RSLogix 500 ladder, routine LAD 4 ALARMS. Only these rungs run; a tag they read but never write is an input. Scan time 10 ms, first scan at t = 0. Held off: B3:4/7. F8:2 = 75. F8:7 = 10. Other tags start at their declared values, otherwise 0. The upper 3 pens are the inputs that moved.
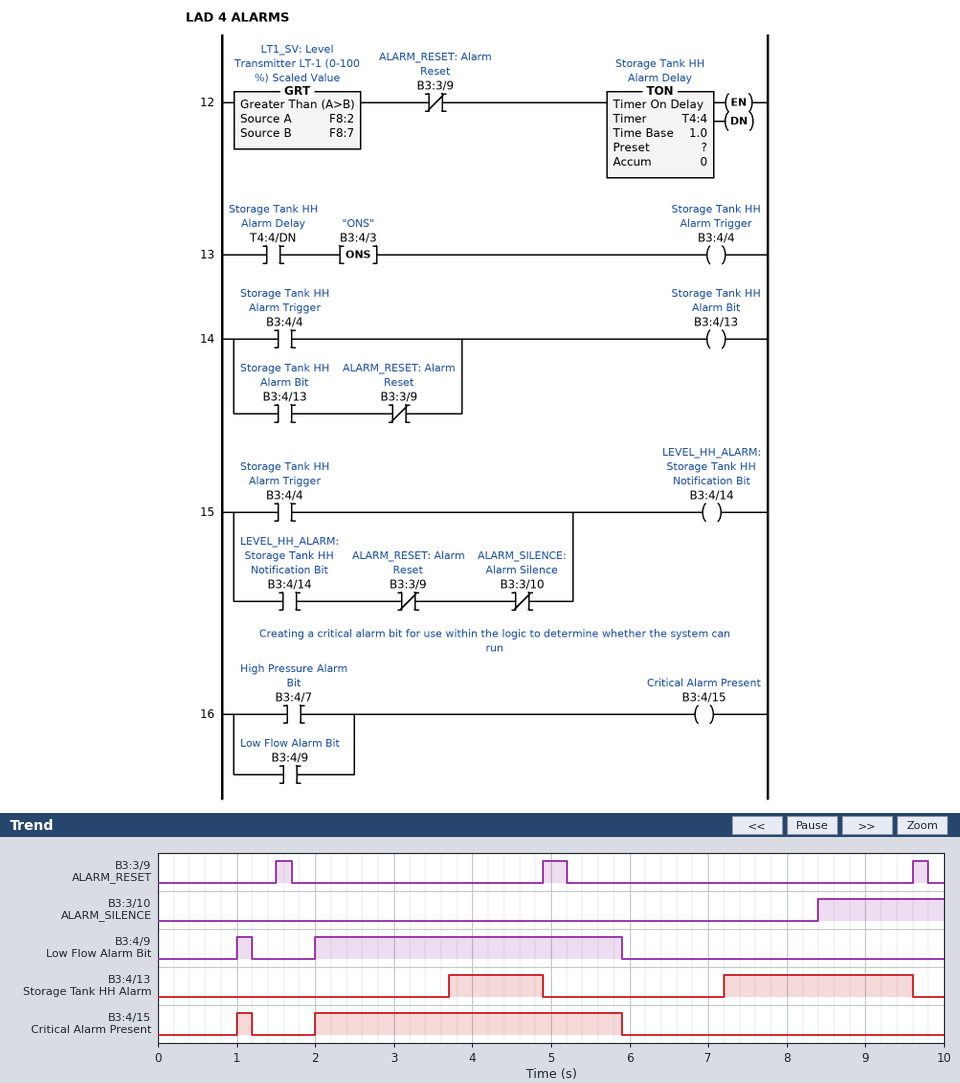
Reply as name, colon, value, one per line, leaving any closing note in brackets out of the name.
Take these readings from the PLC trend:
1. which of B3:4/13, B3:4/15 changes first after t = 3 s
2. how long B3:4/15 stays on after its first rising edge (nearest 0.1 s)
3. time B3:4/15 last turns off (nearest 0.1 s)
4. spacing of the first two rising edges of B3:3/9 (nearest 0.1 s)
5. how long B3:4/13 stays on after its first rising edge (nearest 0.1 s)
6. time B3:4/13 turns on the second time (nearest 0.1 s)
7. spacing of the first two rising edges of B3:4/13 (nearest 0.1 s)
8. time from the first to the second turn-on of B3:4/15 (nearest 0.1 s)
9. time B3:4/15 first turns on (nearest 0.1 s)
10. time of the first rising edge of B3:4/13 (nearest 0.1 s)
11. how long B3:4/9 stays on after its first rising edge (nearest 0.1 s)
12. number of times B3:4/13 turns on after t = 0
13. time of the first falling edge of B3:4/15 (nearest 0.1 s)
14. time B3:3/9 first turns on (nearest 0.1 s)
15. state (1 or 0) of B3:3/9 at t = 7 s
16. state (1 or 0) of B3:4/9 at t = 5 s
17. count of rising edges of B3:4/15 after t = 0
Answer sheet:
which of B3:4/13, B3:4/15 changes first after t = 3 s: B3:4/13
how long B3:4/15 stays on after its first rising edge: 0.2 s
time B3:4/15 last turns off: 5.9 s
spacing of the first two rising edges of B3:3/9: 3.4 s
how long B3:4/13 stays on after its first rising edge: 1.2 s
time B3:4/13 turns on the second time: 7.2 s
spacing of the first two rising edges of B3:4/13: 3.5 s
time from the first to the second turn-on of B3:4/15: 1.0 s
time B3:4/15 first turns on: 1.0 s
time of the first rising edge of B3:4/13: 3.7 s
how long B3:4/9 stays on after its first rising edge: 0.2 s
number of times B3:4/13 turns on after t = 0: 2
time of the first falling edge of B3:4/15: 1.2 s
time B3:3/9 first turns on: 1.5 s
state (1 or 0) of B3:3/9 at t = 7 s: 0
state (1 or 0) of B3:4/9 at t = 5 s: 1
count of rising edges of B3:4/15 after t = 0: 2
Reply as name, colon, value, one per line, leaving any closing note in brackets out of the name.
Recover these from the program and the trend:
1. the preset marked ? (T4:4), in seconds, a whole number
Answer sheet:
the preset marked ? (T4:4), in seconds, a whole number: 2 s
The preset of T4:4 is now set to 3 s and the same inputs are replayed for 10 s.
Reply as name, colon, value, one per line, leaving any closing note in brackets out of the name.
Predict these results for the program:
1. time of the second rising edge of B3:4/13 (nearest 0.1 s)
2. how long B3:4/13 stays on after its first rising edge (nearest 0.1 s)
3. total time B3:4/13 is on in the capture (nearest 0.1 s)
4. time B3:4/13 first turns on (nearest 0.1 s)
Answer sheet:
time of the second rising edge of B3:4/13: 8.2 s
how long B3:4/13 stays on after its first rising edge: 0.2 s
total time B3:4/13 is on in the capture: 1.6 s
time B3:4/13 first turns on: 4.7 s
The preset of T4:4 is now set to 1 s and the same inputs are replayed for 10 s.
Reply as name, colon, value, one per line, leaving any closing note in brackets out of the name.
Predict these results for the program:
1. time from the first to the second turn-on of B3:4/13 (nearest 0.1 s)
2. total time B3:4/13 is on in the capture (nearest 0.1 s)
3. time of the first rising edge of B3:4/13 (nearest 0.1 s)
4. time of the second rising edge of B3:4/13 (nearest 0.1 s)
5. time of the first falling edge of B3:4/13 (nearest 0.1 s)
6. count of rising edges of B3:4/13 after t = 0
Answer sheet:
time from the first to the second turn-on of B3:4/13: 1.7 s
total time B3:4/13 is on in the capture: 6.1 s
time of the first rising edge of B3:4/13: 1.0 s
time of the second rising edge of B3:4/13: 2.7 s
time of the first falling edge of B3:4/13: 1.5 s
count of rising edges of B3:4/13 after t = 0: 3
